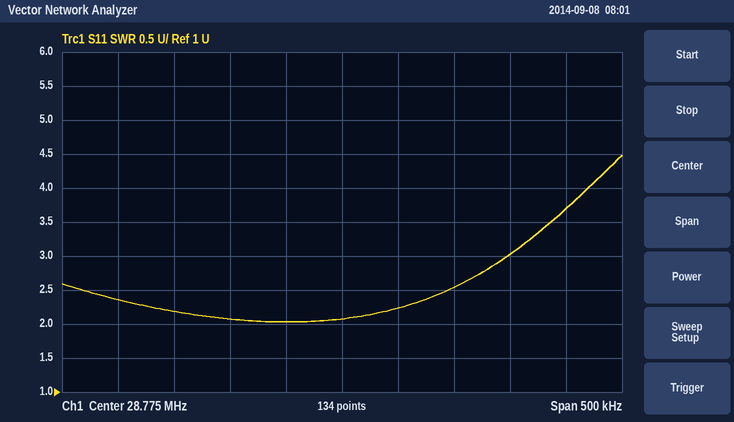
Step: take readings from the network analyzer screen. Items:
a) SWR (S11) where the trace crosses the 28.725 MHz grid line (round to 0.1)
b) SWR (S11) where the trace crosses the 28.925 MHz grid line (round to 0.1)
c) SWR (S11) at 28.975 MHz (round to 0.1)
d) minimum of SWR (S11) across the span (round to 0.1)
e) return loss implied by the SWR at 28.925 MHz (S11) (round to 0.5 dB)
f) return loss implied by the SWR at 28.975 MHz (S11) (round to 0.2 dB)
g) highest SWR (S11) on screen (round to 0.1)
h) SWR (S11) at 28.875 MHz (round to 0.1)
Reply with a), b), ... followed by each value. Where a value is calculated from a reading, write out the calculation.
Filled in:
a) 2.0
b) 3.0
c) 3.7
d) 2.0
e) −20 log10((3 − 1)/(3 + 1)) ≈ 6.0 dB
f) −20 log10((3.7 − 1)/(3.7 + 1)) ≈ 4.8 dB
g) 4.5
h) 2.5
